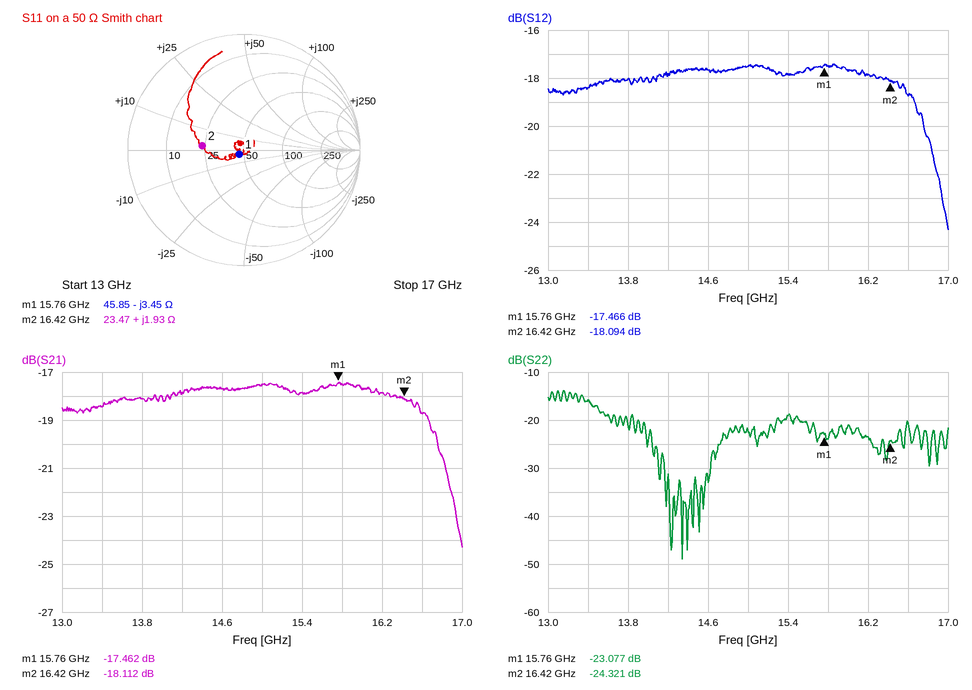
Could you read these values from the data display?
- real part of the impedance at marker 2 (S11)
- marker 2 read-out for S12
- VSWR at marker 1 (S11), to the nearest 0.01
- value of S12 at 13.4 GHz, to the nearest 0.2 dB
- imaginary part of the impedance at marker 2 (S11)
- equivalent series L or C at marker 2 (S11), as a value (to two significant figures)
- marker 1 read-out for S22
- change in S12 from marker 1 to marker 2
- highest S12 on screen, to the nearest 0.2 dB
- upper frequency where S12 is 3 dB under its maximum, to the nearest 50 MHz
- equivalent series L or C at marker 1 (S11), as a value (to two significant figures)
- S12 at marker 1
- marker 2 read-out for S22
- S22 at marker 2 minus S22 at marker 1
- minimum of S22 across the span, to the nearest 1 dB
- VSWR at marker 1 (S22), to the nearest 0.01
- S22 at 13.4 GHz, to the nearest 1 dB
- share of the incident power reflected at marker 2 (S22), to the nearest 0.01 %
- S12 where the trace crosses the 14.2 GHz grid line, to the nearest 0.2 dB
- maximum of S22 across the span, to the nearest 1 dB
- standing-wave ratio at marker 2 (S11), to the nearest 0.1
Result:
23.47 Ω
-18.094 dB
1.12
-18.4 dB
+1.93 Ω
19 pH
-23.077 dB
-0.628 dB
-17.4 dB
16.80 GHz
2.9 pF
-17.466 dB
-24.321 dB
-1.244 dB
-49 dB
1.15
-16 dB
0.37 %
-17.8 dB
-14 dB
2.1
